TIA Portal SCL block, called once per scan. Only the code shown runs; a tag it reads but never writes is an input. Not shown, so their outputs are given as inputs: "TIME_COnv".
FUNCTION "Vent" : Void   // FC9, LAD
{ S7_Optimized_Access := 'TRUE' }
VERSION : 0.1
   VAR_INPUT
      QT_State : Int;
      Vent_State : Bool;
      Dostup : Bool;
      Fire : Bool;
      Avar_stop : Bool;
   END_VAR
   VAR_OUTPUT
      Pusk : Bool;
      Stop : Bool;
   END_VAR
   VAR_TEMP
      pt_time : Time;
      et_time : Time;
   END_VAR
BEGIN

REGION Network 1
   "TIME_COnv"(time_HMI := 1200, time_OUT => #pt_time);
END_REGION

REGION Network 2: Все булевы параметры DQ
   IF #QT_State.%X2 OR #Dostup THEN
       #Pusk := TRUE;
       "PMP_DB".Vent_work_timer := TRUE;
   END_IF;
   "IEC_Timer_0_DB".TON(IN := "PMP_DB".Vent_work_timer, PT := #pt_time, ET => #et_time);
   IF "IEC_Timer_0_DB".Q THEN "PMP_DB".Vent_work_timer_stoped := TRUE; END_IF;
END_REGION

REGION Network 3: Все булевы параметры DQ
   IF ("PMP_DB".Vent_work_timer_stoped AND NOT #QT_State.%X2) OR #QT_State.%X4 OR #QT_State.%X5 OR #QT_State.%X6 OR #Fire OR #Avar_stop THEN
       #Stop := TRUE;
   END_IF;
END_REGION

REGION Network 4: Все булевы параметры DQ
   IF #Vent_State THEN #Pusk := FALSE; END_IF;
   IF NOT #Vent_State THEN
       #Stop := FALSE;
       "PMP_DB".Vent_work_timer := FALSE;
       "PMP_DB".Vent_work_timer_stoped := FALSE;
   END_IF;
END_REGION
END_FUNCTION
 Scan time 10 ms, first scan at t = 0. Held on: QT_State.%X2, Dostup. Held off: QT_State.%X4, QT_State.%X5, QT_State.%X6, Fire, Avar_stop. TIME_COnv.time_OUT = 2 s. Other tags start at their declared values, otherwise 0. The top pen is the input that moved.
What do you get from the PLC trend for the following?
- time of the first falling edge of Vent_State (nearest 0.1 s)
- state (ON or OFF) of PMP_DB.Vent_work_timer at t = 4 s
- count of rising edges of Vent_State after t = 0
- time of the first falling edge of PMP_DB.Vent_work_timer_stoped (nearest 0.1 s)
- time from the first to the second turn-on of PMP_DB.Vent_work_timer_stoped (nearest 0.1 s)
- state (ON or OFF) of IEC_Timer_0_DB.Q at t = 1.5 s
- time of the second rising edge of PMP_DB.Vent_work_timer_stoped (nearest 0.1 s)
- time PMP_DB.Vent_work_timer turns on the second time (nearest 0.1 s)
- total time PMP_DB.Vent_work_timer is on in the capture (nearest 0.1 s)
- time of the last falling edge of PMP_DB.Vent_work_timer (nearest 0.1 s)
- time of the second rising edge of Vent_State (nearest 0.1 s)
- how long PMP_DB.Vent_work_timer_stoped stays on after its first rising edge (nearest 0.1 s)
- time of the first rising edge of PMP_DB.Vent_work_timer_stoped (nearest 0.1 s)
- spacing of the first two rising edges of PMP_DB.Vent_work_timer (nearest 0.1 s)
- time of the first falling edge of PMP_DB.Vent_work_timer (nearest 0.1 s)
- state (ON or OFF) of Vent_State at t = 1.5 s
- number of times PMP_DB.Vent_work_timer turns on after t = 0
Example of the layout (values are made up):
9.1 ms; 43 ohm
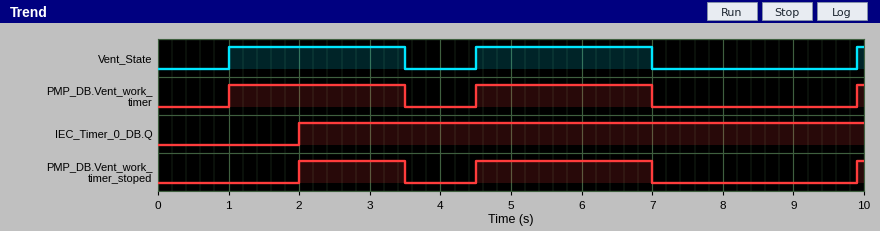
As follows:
3.5 s; OFF; 3; 3.5 s; 2.5 s; OFF; 4.5 s; 4.5 s; 5.1 s; 7.0 s; 4.5 s; 1.5 s; 2.0 s; 3.5 s; 3.5 s; ON; 3
